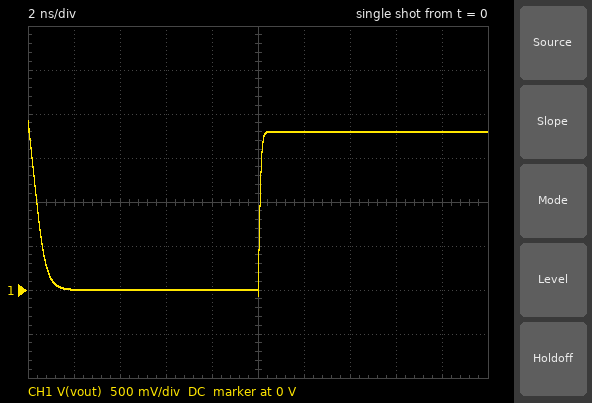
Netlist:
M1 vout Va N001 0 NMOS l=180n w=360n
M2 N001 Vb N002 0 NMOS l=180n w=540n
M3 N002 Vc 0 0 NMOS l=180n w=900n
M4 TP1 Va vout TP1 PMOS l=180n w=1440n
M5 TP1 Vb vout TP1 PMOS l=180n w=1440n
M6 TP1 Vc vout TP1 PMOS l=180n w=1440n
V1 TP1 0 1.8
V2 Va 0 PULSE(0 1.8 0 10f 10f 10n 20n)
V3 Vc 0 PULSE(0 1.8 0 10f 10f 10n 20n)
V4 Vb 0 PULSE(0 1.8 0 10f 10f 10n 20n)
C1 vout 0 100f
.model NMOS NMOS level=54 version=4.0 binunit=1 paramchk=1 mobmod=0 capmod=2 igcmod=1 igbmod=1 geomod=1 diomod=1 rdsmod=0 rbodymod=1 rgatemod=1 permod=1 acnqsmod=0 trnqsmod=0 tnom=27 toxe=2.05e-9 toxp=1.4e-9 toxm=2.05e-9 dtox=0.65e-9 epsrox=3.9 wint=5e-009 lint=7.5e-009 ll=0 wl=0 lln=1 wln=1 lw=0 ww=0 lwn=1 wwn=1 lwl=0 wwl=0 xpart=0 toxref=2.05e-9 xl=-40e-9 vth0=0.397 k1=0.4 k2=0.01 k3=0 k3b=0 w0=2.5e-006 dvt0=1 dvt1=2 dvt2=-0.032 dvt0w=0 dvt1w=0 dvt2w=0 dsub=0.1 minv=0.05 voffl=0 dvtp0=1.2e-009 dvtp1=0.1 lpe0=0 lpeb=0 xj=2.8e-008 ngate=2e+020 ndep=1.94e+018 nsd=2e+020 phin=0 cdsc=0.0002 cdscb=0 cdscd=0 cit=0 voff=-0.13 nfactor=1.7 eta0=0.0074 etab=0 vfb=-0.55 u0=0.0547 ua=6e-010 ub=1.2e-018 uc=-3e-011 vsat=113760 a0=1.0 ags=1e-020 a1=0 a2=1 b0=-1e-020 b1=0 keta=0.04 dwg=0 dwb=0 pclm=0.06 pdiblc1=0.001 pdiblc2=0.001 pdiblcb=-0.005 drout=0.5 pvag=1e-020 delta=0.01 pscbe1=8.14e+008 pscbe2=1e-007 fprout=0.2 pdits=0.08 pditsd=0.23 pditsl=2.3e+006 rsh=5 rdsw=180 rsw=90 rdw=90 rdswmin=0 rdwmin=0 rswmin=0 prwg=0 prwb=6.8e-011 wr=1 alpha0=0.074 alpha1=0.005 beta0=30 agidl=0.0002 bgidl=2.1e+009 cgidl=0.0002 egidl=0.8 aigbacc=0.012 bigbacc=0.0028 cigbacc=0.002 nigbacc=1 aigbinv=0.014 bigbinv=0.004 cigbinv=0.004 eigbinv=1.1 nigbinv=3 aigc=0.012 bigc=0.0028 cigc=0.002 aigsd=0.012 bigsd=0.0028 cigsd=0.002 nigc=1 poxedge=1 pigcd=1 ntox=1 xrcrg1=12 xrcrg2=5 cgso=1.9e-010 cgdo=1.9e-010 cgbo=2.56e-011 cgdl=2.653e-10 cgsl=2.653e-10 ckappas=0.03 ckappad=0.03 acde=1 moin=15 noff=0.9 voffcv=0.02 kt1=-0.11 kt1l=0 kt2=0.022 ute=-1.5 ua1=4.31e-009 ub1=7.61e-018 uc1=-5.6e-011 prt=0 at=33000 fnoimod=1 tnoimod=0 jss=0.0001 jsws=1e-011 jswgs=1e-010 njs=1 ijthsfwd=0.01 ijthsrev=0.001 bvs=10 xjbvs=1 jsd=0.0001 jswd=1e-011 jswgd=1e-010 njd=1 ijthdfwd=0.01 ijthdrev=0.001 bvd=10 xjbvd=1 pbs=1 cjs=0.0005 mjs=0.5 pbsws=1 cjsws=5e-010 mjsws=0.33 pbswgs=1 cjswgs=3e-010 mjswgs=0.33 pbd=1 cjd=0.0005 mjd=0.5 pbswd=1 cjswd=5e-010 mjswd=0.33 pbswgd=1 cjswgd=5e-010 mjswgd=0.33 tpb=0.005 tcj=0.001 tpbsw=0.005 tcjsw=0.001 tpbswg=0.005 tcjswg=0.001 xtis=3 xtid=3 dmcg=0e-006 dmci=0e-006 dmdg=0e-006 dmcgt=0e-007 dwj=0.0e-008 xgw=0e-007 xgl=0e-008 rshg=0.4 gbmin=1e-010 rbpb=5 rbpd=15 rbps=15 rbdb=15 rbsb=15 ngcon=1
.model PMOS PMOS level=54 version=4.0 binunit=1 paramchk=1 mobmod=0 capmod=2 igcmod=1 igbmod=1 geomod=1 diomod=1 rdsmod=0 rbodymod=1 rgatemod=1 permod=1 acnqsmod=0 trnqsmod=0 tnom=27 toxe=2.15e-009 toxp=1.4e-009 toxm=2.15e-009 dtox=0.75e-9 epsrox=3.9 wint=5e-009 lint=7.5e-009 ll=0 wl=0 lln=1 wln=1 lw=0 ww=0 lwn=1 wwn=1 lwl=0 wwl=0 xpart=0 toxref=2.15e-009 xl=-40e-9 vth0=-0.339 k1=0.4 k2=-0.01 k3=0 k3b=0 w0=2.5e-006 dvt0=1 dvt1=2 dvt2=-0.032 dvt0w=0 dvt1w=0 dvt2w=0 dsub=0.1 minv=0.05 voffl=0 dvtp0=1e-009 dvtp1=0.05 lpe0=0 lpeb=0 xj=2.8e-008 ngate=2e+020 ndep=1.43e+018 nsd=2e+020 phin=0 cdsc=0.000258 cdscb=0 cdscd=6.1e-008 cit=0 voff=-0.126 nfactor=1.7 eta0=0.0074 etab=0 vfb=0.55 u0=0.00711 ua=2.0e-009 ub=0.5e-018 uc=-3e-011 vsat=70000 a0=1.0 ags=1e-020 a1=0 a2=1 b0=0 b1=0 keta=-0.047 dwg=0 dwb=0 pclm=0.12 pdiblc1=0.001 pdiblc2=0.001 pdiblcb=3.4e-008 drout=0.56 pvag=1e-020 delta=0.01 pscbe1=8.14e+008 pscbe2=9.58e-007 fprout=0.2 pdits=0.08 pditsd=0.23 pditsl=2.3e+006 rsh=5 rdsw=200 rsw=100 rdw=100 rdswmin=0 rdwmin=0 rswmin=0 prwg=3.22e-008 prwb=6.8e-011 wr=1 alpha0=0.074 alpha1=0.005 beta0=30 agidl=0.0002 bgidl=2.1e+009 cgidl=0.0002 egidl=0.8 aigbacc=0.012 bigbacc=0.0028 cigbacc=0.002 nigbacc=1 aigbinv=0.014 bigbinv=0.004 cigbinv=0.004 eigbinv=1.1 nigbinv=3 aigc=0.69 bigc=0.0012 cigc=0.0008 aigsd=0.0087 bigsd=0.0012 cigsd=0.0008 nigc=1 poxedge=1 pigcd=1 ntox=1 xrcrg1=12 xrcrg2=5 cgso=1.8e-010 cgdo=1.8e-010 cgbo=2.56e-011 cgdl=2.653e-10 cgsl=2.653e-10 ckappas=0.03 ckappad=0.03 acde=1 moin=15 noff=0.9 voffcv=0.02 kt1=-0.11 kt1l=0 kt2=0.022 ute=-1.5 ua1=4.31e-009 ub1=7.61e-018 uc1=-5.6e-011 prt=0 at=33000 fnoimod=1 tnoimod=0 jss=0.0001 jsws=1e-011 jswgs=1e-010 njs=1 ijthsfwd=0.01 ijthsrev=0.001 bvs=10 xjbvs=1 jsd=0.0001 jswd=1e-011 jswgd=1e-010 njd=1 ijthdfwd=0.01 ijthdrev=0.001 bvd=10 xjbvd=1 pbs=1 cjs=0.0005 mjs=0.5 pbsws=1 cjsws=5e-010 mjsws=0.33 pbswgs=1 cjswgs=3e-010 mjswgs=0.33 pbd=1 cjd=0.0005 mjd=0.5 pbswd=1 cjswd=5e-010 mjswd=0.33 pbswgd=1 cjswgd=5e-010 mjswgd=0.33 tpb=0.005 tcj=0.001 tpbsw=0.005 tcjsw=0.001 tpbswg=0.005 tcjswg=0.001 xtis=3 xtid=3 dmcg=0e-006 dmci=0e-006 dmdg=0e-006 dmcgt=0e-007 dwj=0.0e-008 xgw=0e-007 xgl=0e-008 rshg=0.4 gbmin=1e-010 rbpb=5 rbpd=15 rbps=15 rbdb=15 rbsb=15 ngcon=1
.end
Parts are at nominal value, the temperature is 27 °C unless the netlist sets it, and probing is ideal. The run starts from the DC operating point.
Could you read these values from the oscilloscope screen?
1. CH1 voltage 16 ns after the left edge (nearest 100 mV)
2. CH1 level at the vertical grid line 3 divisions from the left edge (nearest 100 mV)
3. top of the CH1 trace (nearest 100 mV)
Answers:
1.8 V
0 V
1.9 V
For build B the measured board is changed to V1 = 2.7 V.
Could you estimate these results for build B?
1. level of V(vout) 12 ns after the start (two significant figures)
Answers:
2.7 V
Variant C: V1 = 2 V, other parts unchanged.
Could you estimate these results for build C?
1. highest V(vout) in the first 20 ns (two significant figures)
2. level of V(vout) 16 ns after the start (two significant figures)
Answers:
2.1 V
2.0 V
